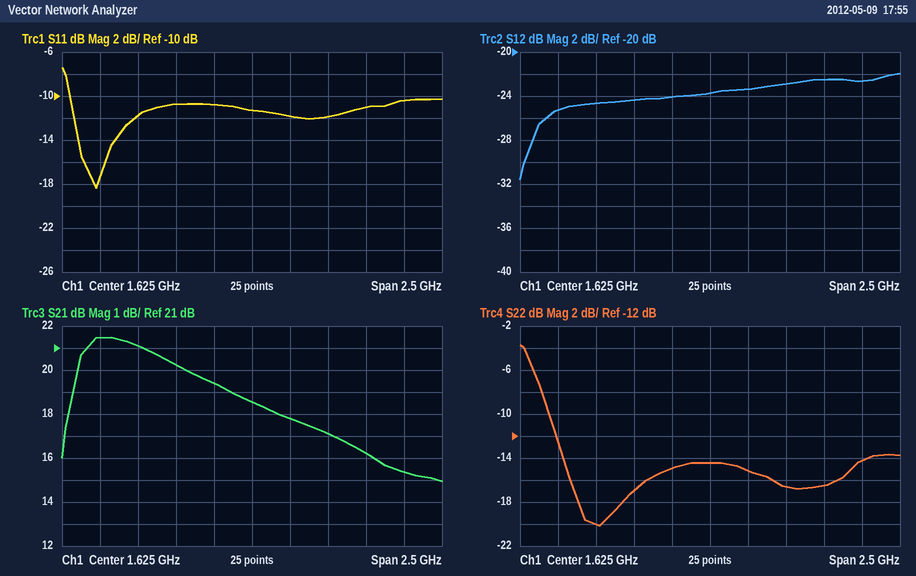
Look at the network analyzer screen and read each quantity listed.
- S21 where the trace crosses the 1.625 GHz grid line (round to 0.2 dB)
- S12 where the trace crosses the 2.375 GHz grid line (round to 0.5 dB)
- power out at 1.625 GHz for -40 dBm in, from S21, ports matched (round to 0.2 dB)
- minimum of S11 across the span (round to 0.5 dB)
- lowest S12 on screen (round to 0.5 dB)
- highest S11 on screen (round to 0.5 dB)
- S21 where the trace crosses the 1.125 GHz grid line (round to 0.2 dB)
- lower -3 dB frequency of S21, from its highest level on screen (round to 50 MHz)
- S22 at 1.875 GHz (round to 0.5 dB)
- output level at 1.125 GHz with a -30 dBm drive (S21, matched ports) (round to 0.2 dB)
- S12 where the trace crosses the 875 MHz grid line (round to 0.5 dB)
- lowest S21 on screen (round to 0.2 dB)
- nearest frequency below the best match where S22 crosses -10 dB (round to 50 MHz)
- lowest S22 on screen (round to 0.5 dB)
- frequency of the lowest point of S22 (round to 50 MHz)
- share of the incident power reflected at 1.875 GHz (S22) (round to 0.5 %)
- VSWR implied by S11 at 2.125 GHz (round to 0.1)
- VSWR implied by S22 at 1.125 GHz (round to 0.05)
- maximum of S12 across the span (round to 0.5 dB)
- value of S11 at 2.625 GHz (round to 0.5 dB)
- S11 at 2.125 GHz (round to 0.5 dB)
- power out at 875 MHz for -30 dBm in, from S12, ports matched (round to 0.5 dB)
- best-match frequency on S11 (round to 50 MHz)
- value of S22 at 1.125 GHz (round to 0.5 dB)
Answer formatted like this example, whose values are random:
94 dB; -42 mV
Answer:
18.6 dB; -22.5 dB; -21.4 dBm; -18.5 dB; -31.5 dB; -7.5 dB; 20.2 dB; 450 MHz; -15.0 dB; -9.8 dBm; -24.5 dB; 15.0 dB; 550 MHz; -20.0 dB; 900 MHz; 3.0 %; 1.7; 1.35; -22.0 dB; -10.5 dB; -12.0 dB; -54.5 dBm; 600 MHz; -17.0 dB
